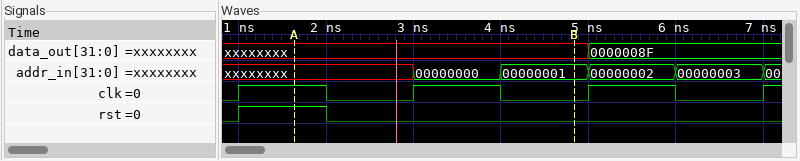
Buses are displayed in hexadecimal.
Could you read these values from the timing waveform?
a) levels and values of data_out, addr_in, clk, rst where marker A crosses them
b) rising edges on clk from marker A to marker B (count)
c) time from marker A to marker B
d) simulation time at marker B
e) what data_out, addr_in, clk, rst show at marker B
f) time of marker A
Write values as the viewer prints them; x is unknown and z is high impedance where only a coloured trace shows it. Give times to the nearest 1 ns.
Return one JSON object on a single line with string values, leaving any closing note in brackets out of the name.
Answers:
{"levels and values of data_out, addr_in, clk, rst where marker A crosses them": "data_out=xxxxxxxx, addr_in=xxxxxxxx, clk=1, rst=1", "rising edges on clk from marker A to marker B": "1", "time from marker A to marker B": "3 ns", "simulation time at marker B": "5 ns", "what data_out, addr_in, clk, rst show at marker B": "data_out=xxxxxxxx, addr_in=00000001, clk=0, rst=0", "time of marker A": "2 ns"}
